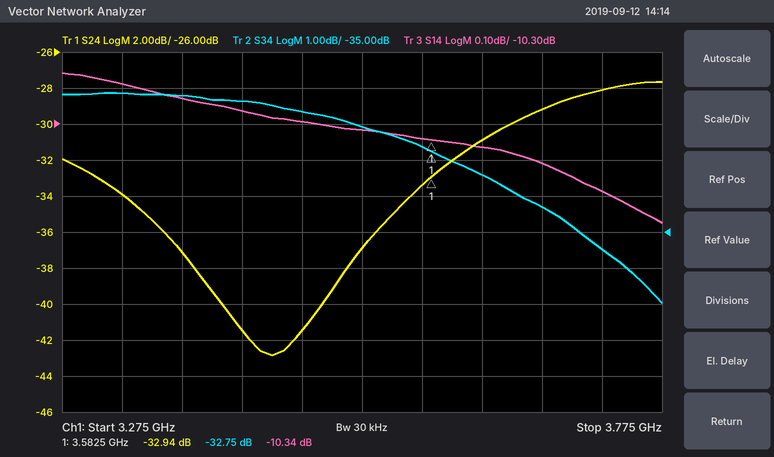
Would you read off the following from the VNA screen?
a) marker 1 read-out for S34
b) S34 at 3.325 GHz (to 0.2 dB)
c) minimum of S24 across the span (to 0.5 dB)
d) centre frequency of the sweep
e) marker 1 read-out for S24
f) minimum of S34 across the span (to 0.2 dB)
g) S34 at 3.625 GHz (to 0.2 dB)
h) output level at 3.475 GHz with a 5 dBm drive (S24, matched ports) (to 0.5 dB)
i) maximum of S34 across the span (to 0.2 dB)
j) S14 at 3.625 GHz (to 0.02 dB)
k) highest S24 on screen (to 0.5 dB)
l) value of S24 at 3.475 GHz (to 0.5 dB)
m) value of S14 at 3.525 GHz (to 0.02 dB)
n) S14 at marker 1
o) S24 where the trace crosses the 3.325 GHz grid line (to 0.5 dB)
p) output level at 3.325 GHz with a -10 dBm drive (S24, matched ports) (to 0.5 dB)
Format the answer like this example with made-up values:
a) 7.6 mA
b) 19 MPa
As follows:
a) -32.75 dB
b) -31.2 dB
c) -43.0 dB
d) 3.525 GHz
e) -32.94 dB
f) -37.0 dB
g) -33.4 dB
h) -36.5 dBm
i) -31.2 dB
j) -10.36 dB
k) -27.5 dB
l) -41.5 dB
m) -10.32 dB
n) -10.34 dB
o) -34.0 dB
p) -44.0 dBm
